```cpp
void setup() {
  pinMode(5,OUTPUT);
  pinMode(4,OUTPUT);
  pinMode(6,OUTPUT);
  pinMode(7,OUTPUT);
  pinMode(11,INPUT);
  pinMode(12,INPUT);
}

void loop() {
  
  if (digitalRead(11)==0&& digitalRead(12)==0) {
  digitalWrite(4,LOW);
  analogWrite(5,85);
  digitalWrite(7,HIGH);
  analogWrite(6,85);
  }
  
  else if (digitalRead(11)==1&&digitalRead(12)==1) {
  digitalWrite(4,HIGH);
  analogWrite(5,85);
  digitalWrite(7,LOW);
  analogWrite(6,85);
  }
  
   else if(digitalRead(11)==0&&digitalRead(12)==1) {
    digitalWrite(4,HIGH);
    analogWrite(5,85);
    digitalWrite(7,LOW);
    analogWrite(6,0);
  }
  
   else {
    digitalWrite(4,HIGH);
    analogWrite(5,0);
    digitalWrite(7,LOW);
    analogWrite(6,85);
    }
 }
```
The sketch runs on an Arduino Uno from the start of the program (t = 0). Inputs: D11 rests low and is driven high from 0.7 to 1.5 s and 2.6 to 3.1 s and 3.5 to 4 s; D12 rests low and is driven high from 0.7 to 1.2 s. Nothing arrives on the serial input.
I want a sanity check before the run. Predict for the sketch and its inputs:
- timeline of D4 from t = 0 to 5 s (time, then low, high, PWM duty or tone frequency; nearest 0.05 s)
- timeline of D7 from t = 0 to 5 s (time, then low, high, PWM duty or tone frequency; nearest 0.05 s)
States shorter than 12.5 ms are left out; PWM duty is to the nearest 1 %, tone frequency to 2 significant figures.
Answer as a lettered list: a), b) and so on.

a) 0 s low; 0.7 s high; 1.5 s low; 2.6 s high; 3.1 s low; 3.5 s high; 4 s low
b) 0 s high; 0.7 s low; 1.5 s high; 2.6 s low; 3.1 s high; 3.5 s low; 4 s high
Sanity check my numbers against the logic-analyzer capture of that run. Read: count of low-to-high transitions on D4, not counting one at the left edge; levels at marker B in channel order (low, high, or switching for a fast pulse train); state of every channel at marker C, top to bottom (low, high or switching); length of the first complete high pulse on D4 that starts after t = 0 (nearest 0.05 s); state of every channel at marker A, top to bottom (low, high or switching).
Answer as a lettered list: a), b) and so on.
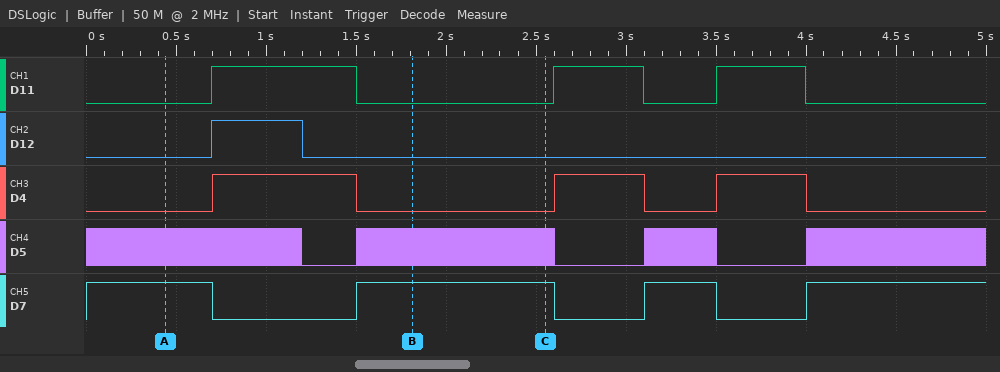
a) 3
b) D11 low, D12 low, D4 low, D5 switching, D7 high
c) D11 low, D12 low, D4 low, D5 switching, D7 high
d) 0.80 s
e) D11 low, D12 low, D4 low, D5 switching, D7 high
